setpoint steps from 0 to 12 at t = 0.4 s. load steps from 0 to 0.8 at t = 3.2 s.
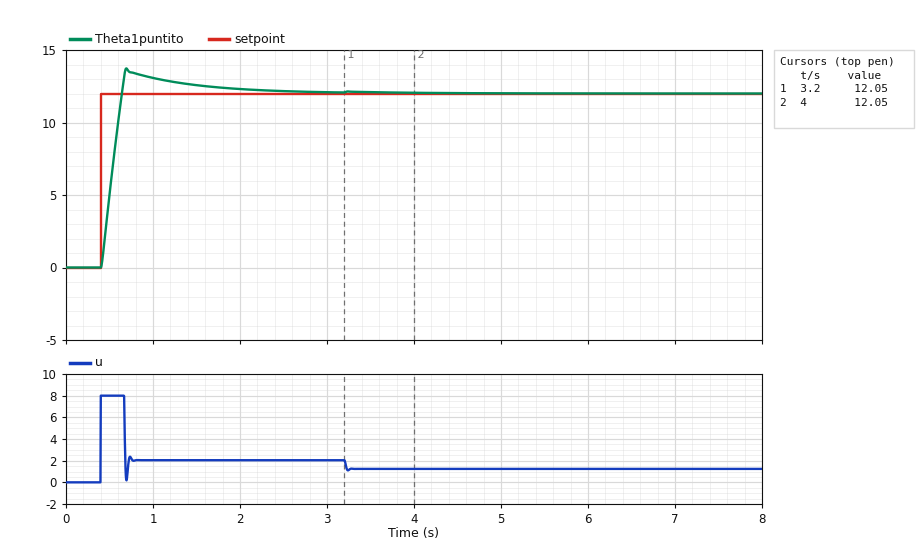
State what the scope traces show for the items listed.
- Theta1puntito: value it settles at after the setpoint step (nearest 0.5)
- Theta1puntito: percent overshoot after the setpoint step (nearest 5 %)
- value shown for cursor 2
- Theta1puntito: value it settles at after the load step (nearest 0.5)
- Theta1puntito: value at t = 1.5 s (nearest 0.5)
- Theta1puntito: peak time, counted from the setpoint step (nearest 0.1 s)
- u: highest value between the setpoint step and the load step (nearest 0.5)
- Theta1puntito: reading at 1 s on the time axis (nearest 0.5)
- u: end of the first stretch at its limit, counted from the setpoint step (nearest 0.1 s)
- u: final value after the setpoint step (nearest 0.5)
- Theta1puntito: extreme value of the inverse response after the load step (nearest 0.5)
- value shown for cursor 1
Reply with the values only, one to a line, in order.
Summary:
12.0
15 %
12.05
12.0
12.5
0.3 s
8.0
13.0
0.3 s
2.0
12.0
12.05
